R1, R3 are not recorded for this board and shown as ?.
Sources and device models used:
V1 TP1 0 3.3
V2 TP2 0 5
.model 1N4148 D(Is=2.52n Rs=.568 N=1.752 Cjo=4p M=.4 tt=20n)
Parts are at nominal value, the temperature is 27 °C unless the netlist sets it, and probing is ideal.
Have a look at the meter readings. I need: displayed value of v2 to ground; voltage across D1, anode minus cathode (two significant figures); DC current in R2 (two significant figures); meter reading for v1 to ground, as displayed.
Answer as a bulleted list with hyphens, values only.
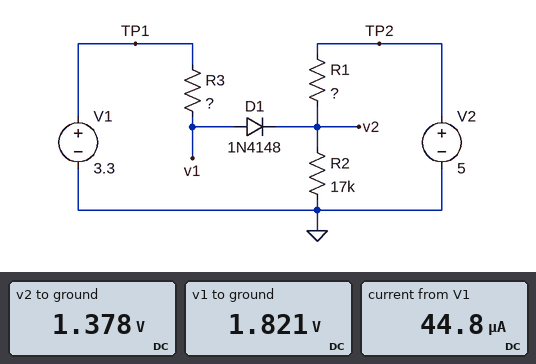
- 1.378 V
- 440 mV
- 81 µA
- 1.821 V
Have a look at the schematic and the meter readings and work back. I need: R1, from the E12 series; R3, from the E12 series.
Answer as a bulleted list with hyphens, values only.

- 100 kΩ
- 33 kΩ
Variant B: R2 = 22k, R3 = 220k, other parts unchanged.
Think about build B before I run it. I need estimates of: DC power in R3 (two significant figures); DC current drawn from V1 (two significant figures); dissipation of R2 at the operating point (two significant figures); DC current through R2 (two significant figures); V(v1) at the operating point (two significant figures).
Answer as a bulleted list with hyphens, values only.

- 16 µW
- 8.5 µA
- 51 µW
- 48 µA
- 1.4 V
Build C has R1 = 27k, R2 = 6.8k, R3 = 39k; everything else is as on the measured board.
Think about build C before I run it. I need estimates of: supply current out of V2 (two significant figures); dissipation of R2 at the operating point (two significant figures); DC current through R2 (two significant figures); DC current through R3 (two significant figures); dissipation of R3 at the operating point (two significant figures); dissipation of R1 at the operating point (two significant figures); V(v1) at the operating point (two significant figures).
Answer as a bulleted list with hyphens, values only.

- 140 µA
- 220 µW
- 180 µA
- 42 µA
- 68 µW
- 530 µW
- 1.7 V
